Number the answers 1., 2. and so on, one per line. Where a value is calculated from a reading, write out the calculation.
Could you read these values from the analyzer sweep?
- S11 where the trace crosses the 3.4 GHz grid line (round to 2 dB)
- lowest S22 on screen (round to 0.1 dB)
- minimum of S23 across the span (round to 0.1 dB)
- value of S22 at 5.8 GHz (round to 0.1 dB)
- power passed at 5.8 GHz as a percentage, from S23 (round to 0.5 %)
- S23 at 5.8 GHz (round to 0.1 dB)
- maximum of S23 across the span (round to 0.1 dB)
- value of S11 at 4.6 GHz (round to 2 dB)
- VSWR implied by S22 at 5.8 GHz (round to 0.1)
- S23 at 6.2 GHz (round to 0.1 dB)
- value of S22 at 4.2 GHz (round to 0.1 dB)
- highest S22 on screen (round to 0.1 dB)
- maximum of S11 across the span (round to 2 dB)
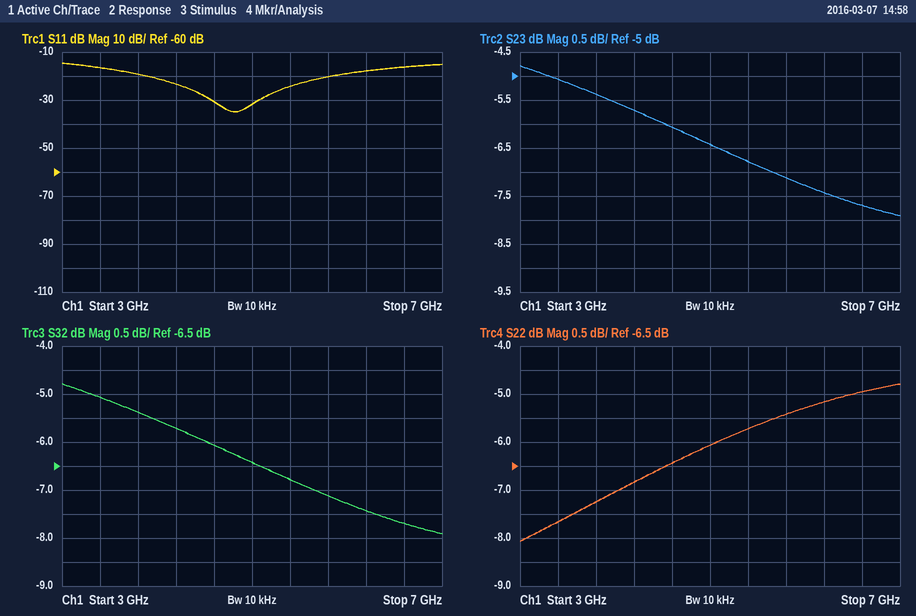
1. -16 dB
2. -8.1 dB
3. -7.9 dB
4. -5.4 dB
5. 10^(-7.1/10) ≈ 19.5 %
6. -7.1 dB
7. -4.8 dB
8. -30 dB
9. |Γ| = 10^(-5.4/20) = 0.5370; VSWR = (1 + 0.5370)/(1 − 0.5370) ≈ 3.3
10. -7.4 dB
11. -6.8 dB
12. -4.8 dB
13. -14 dB
